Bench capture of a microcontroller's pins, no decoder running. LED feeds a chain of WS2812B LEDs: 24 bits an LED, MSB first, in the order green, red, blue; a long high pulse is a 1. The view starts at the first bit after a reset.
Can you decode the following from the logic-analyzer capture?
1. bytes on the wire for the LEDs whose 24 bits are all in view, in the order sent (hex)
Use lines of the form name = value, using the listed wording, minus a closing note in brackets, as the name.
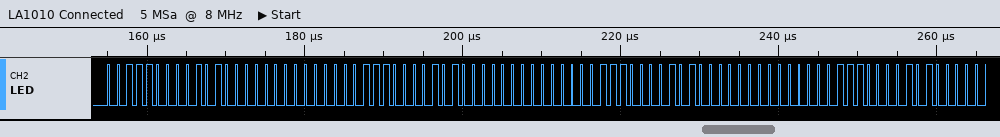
bytes on the wire for the LEDs whose 24 bits are all in view, in the order sent = 38 50 00 38 50 00 38 50 00
